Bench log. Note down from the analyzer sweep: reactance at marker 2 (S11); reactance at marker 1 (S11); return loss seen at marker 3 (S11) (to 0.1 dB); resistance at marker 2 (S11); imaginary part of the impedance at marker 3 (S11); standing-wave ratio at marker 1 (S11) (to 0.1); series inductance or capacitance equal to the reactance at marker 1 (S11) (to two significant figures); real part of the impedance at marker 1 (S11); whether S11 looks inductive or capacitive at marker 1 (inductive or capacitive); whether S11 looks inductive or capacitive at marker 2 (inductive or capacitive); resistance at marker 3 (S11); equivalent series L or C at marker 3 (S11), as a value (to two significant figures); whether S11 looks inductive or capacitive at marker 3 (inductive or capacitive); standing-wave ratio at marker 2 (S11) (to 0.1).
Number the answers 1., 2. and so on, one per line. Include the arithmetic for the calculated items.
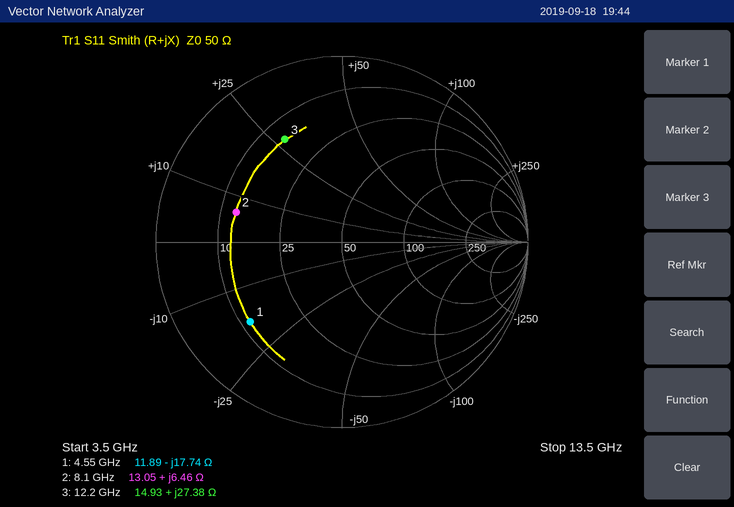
1. +6.46 Ω
2. -17.74 Ω
3. 4.0 dB
4. 13.05 Ω
5. +27.38 Ω
6. 4.8
7. C = 1/(2π × 4.55 GHz × 17.74 Ω) ≈ 2.0 pF
8. 11.89 Ω
9. capacitive
10. inductive
11. 14.93 Ω
12. L = 27.38 Ω/(2π × 12.2 GHz) ≈ 357 pH, so 360 pH to two significant figures
13. inductive
14. 3.9
